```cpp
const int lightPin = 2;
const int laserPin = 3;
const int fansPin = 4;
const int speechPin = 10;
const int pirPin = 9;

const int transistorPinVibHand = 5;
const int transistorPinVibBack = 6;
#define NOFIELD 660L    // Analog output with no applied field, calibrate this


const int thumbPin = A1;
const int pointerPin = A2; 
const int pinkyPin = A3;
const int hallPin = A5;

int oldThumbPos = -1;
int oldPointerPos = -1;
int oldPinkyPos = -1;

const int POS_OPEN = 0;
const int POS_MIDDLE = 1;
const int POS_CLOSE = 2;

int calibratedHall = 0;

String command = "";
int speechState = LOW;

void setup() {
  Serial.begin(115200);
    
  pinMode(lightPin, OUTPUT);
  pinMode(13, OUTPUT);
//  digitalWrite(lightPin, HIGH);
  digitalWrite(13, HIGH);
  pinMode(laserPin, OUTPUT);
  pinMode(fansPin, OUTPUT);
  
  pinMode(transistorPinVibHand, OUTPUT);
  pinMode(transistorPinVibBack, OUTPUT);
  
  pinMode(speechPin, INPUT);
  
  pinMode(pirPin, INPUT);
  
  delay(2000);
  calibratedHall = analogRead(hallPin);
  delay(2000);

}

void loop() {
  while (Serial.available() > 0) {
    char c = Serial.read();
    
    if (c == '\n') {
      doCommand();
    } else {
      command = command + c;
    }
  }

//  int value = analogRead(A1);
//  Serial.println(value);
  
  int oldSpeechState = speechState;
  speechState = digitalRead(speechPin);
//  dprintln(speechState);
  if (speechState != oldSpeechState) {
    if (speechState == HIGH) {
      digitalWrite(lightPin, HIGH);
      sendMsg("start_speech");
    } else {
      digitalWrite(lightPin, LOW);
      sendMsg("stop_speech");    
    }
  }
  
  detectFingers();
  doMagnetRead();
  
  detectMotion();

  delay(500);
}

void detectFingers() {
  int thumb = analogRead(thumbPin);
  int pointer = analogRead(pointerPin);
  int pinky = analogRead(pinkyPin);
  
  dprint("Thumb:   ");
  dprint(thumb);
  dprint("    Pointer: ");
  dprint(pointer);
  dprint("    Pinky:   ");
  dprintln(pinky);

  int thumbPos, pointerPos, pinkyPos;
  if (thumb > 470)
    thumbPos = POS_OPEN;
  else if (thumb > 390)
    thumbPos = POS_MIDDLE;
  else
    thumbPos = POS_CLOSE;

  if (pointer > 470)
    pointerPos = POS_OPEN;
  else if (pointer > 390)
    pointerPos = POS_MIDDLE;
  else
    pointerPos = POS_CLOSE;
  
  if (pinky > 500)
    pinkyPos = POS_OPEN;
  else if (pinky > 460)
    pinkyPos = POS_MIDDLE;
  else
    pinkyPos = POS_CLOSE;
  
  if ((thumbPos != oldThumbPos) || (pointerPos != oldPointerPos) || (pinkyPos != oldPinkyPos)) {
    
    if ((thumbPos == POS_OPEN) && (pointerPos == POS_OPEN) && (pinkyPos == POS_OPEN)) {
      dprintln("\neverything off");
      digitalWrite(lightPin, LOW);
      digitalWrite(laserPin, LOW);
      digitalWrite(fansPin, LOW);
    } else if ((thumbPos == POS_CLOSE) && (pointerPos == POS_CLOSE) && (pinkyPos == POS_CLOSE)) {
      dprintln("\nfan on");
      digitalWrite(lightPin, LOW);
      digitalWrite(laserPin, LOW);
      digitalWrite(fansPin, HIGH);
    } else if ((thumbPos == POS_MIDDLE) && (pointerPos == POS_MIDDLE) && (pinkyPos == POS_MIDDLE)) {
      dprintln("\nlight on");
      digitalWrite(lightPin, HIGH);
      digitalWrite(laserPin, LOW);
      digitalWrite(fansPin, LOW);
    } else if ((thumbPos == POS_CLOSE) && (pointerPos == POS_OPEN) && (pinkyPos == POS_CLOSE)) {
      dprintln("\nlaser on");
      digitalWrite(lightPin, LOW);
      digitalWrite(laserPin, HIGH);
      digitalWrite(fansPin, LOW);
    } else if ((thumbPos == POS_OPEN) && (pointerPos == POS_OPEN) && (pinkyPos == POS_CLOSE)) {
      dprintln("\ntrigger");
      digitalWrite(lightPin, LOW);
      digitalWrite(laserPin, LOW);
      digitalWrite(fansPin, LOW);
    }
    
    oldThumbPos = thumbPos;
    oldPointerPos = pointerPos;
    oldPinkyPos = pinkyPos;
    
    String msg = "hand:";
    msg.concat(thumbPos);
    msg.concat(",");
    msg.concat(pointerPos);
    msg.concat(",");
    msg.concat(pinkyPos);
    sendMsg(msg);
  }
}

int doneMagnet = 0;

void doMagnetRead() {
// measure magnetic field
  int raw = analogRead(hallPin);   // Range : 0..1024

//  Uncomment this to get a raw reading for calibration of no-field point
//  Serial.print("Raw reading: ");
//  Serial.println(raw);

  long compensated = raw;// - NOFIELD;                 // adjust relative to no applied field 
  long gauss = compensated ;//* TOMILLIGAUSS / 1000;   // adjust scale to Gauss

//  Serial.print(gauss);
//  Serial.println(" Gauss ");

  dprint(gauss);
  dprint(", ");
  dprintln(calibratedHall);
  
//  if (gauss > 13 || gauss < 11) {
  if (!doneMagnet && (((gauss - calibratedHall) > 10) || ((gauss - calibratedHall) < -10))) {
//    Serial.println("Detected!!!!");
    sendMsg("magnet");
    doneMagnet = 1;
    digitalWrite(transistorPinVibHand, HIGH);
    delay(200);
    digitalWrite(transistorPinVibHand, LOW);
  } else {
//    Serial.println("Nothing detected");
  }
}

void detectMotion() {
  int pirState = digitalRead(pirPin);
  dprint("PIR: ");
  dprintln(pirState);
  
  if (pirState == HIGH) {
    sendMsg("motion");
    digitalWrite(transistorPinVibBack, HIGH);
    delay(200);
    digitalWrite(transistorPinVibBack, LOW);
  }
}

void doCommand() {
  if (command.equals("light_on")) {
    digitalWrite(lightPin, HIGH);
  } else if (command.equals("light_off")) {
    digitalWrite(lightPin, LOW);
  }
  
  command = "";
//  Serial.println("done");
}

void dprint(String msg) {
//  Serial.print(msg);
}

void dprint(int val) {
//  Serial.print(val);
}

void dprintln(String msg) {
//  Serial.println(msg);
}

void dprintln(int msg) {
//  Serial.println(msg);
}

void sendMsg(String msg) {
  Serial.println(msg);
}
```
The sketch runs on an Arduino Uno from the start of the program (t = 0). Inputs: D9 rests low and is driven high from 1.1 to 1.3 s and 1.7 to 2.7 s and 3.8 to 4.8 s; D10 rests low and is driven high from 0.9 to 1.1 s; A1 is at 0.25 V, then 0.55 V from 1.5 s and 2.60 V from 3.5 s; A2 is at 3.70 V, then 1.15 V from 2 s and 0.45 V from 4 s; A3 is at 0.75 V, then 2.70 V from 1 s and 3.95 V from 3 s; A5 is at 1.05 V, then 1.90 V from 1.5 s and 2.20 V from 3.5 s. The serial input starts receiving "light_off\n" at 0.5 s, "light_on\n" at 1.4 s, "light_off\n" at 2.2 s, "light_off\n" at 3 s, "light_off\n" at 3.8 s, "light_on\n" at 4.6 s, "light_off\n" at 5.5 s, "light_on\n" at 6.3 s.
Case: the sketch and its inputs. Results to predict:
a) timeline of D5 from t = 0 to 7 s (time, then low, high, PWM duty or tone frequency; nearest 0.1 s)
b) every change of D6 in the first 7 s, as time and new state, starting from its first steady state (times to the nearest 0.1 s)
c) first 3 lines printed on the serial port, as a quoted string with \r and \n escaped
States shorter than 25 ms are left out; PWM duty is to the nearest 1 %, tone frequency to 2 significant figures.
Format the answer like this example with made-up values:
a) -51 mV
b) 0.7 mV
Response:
a) 0 s low; 4 s high; 4.2 s low
b) 0 s low; 4.2 s high; 4.4 s low
c) "hand:0,2,0\r\nmagnet\r\nmotion\r\n"
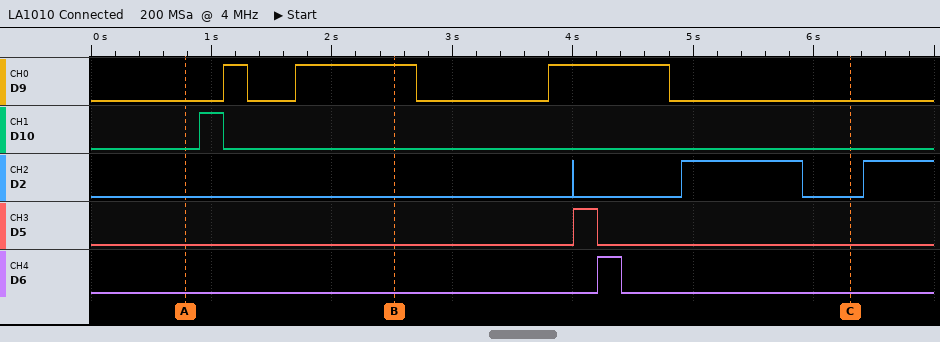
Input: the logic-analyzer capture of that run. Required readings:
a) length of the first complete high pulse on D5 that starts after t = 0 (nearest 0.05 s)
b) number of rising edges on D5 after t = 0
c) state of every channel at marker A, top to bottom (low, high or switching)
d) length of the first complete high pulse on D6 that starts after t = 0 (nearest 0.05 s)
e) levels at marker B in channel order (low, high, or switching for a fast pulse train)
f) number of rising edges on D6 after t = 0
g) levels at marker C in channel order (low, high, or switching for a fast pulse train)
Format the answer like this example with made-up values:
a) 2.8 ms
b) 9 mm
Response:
a) 0.20 s
b) 1
c) D9 low, D10 low, D2 low, D5 low, D6 low
d) 0.20 s
e) D9 high, D10 low, D2 low, D5 low, D6 low
f) 1
g) D9 low, D10 low, D2 low, D5 low, D6 low
